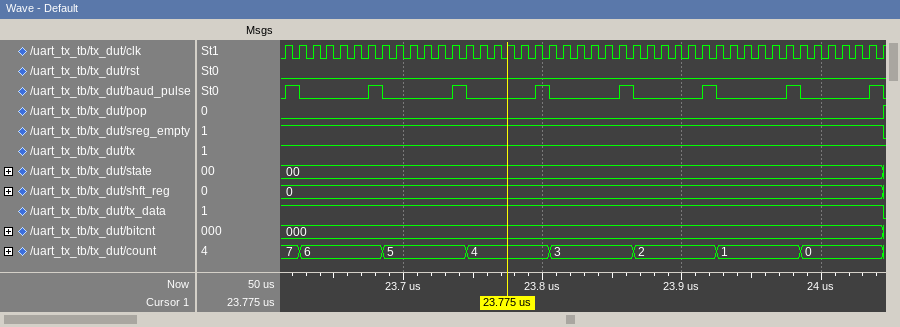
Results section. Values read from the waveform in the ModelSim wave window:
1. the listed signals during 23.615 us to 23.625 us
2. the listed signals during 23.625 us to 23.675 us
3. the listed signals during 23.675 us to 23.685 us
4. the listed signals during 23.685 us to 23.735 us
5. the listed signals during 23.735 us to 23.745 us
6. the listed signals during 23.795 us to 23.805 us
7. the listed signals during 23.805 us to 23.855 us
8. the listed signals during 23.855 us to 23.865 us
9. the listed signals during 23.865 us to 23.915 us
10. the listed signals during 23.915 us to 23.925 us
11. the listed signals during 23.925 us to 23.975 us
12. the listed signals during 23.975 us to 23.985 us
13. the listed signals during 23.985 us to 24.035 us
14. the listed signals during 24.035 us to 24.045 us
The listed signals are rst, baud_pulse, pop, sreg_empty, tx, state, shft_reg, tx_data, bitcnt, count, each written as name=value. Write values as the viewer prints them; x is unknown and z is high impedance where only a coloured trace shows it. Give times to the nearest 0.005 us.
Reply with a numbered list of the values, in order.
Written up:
1. rst=0, baud_pulse=1, pop=0, sreg_empty=1, tx=1, state=00, shft_reg=0, tx_data=1, bitcnt=000, count=7
2. rst=0, baud_pulse=0, pop=0, sreg_empty=1, tx=1, state=00, shft_reg=0, tx_data=1, bitcnt=000, count=6
3. rst=0, baud_pulse=1, pop=0, sreg_empty=1, tx=1, state=00, shft_reg=0, tx_data=1, bitcnt=000, count=6
4. rst=0, baud_pulse=0, pop=0, sreg_empty=1, tx=1, state=00, shft_reg=0, tx_data=1, bitcnt=000, count=5
5. rst=0, baud_pulse=1, pop=0, sreg_empty=1, tx=1, state=00, shft_reg=0, tx_data=1, bitcnt=000, count=5
6. rst=0, baud_pulse=1, pop=0, sreg_empty=1, tx=1, state=00, shft_reg=0, tx_data=1, bitcnt=000, count=4
7. rst=0, baud_pulse=0, pop=0, sreg_empty=1, tx=1, state=00, shft_reg=0, tx_data=1, bitcnt=000, count=3
8. rst=0, baud_pulse=1, pop=0, sreg_empty=1, tx=1, state=00, shft_reg=0, tx_data=1, bitcnt=000, count=3
9. rst=0, baud_pulse=0, pop=0, sreg_empty=1, tx=1, state=00, shft_reg=0, tx_data=1, bitcnt=000, count=2
10. rst=0, baud_pulse=1, pop=0, sreg_empty=1, tx=1, state=00, shft_reg=0, tx_data=1, bitcnt=000, count=2
11. rst=0, baud_pulse=0, pop=0, sreg_empty=1, tx=1, state=00, shft_reg=0, tx_data=1, bitcnt=000, count=1
12. rst=0, baud_pulse=1, pop=0, sreg_empty=1, tx=1, state=00, shft_reg=0, tx_data=1, bitcnt=000, count=1
13. rst=0, baud_pulse=0, pop=0, sreg_empty=1, tx=1, state=00, shft_reg=0, tx_data=1, bitcnt=000, count=0
14. rst=0, baud_pulse=1, pop=0, sreg_empty=1, tx=1, state=00, shft_reg=0, tx_data=1, bitcnt=000, count=0
